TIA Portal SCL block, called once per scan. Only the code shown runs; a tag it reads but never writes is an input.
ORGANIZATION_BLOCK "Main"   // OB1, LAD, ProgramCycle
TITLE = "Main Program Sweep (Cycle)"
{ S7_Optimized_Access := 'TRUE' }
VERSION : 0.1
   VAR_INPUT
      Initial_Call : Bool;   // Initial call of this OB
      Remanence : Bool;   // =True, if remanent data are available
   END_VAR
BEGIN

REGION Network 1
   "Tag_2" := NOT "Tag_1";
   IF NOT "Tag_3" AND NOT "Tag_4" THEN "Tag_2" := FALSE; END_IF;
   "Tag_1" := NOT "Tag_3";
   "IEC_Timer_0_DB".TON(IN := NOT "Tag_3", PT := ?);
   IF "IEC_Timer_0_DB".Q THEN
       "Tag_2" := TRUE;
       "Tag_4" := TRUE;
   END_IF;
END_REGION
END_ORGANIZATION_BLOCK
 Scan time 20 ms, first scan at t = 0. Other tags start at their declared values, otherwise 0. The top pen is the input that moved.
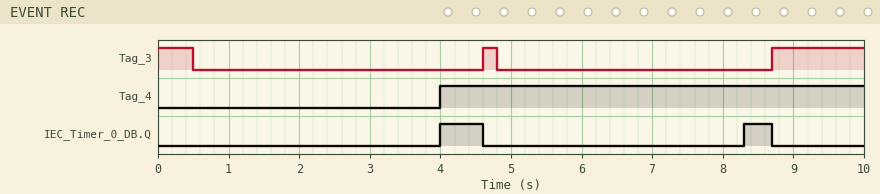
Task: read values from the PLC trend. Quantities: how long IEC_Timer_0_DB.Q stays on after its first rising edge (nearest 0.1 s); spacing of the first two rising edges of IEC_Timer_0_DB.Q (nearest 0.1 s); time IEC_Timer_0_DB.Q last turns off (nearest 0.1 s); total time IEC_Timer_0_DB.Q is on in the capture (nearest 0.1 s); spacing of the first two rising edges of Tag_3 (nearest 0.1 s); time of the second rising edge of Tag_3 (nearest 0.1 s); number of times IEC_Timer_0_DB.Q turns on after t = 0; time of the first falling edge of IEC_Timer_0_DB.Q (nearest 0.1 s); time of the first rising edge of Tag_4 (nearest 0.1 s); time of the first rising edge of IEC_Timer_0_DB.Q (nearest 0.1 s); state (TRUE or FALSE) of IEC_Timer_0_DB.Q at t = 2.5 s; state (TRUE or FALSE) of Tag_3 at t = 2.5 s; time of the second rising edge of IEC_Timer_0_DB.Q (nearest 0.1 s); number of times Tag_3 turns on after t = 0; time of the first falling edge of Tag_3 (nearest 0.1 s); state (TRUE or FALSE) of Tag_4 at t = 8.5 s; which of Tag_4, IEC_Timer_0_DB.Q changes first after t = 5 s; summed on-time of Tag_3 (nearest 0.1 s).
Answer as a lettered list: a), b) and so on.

a) 0.6 s
b) 4.3 s
c) 8.7 s
d) 1.0 s
e) 4.1 s
f) 8.7 s
g) 2
h) 4.6 s
i) 4.0 s
j) 4.0 s
k) FALSE
l) FALSE
m) 8.3 s
n) 2
o) 0.5 s
p) TRUE
q) IEC_Timer_0_DB.Q
r) 2.0 s
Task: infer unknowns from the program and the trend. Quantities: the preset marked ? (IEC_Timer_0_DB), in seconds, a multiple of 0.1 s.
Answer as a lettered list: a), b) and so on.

a) 3.5 s
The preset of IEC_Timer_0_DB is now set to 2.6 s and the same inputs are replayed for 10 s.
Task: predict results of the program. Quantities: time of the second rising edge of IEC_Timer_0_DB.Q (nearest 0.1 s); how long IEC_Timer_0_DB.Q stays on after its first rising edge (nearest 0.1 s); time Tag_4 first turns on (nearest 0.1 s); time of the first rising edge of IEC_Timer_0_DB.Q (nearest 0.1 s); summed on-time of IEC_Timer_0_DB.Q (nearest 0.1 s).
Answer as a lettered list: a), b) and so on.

a) 7.4 s
b) 1.5 s
c) 3.1 s
d) 3.1 s
e) 2.8 s
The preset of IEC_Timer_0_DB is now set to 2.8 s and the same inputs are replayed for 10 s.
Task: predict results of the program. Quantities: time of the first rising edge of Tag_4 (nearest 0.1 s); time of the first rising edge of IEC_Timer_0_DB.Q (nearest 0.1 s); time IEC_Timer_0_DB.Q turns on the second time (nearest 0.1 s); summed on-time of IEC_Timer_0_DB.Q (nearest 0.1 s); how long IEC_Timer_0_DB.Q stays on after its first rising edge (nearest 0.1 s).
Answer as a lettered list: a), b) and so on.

a) 3.3 s
b) 3.3 s
c) 7.6 s
d) 2.4 s
e) 1.3 s
